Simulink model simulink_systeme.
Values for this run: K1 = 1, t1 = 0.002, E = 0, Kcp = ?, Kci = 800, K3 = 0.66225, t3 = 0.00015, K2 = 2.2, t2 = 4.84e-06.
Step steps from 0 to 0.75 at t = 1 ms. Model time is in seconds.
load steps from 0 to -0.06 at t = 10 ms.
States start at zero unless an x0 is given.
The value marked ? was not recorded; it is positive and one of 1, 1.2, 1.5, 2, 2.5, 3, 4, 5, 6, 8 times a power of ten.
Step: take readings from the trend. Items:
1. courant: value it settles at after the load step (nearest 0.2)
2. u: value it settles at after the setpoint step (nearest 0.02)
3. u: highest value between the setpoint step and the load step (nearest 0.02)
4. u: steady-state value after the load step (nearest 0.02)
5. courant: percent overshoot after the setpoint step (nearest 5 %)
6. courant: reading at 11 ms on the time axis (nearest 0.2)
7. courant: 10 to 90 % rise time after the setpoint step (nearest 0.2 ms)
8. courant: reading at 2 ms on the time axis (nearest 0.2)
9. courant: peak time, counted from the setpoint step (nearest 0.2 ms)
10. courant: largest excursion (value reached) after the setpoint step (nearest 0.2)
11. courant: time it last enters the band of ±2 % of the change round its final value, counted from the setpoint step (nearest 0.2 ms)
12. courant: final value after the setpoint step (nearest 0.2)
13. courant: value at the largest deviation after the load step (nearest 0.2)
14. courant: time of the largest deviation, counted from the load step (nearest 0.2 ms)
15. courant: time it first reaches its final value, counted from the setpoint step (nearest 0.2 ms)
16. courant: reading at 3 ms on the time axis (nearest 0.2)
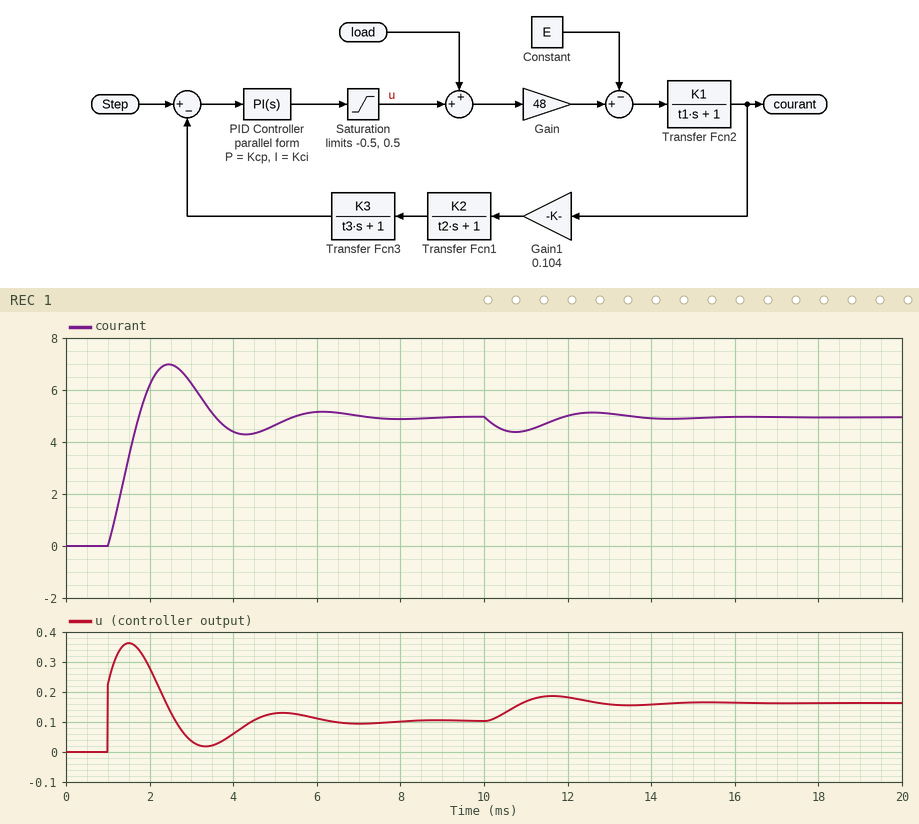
5.0
0.10
0.36
0.16
40 %
4.4
0.6 ms
6.2
1.4 ms
7.0
5.8 ms
5.0
4.4
0.8 ms
0.8 ms
6.2
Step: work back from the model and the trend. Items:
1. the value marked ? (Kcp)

0.3
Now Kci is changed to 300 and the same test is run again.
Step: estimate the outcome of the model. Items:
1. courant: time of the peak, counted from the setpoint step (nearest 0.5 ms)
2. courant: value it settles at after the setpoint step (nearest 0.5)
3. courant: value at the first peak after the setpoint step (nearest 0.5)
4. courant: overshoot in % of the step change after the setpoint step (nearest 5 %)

2.5 ms
5.0
5.5
10 %
